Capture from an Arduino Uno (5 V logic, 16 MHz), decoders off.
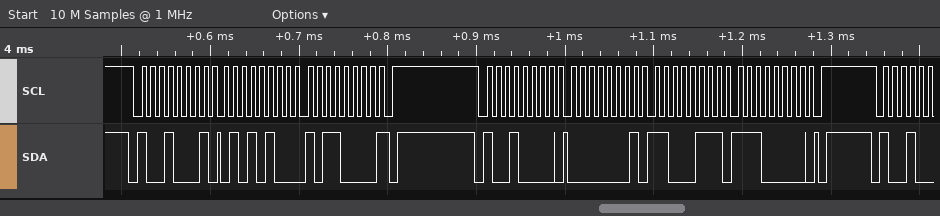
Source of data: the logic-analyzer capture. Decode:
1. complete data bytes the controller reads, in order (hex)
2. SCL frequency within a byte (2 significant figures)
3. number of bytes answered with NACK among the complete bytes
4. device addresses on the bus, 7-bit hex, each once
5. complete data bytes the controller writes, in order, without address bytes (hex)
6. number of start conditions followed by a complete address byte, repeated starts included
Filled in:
54 B0
100 kHz
1
0x48
01 C7 E0
2
